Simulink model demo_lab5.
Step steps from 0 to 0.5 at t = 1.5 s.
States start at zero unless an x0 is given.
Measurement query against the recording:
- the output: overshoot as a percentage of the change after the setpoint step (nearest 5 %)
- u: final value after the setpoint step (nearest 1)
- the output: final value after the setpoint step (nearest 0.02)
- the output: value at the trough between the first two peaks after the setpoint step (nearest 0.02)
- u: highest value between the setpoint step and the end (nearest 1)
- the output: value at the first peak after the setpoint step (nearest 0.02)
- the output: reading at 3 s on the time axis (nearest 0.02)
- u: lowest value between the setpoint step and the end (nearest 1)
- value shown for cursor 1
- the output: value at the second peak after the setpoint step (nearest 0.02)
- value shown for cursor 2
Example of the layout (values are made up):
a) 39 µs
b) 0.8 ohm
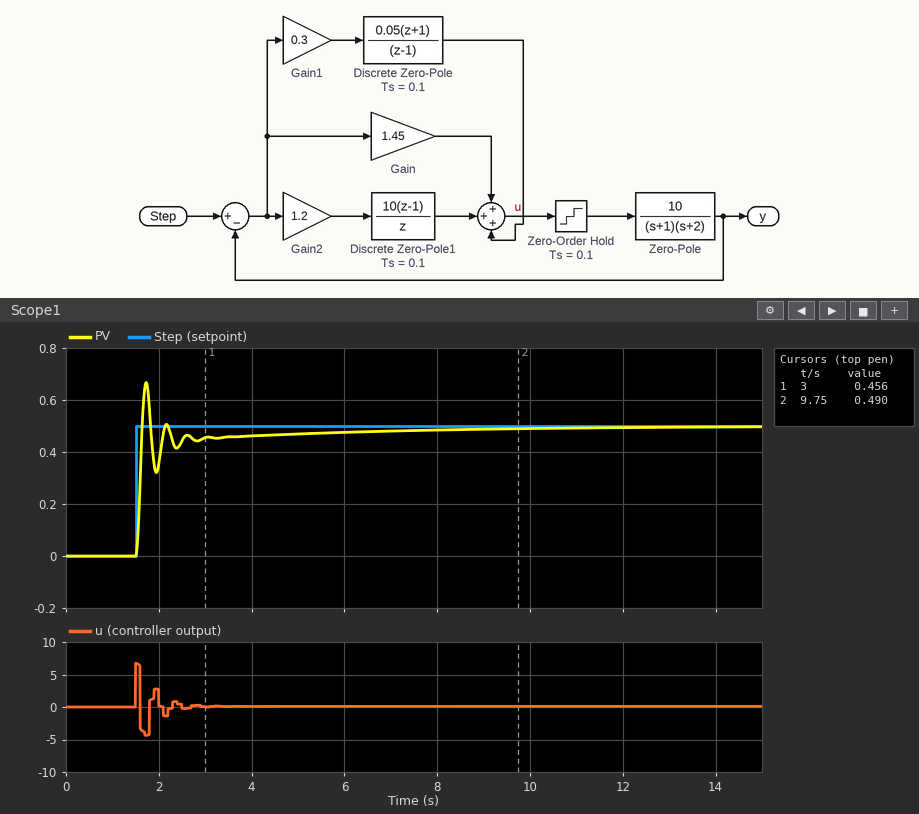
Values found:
a) 35 %
b) 0
c) 0.50
d) 0.32
e) 7
f) 0.66
g) 0.46
h) -4
i) 0.456
j) 0.50
k) 0.490
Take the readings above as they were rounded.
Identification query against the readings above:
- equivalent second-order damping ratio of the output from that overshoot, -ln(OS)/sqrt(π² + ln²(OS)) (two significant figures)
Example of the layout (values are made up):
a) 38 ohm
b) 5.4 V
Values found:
a) 0.32
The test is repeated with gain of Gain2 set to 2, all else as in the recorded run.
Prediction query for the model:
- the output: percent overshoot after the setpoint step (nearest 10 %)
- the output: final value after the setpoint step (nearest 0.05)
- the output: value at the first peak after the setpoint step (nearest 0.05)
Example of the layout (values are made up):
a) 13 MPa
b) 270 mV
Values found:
a) 70 %
b) 0.50
c) 0.85
